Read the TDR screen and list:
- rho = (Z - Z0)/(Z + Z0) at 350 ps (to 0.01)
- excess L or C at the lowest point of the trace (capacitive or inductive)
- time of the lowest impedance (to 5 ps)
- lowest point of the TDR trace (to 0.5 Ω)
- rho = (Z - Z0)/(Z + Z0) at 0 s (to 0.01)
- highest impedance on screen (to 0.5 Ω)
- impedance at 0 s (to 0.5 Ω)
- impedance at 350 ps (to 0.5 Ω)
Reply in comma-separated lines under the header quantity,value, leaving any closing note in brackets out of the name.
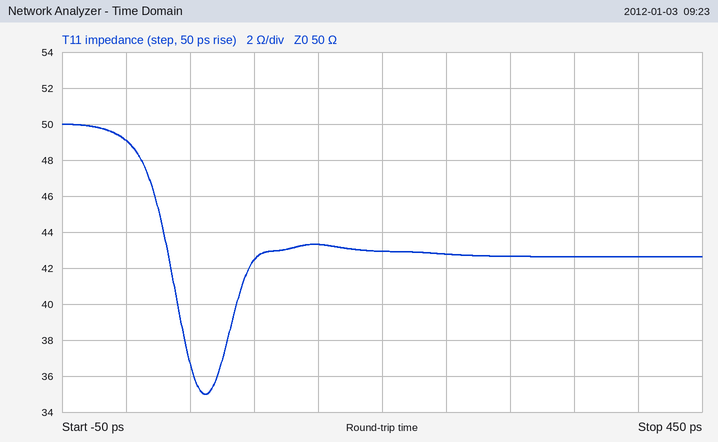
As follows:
quantity,value
rho = (Z - Z0)/(Z + Z0) at 350 ps,-0.08
excess L or C at the lowest point of the trace,capacitive
time of the lowest impedance,60 ps
lowest point of the TDR trace,35.0 Ω
rho = (Z - Z0)/(Z + Z0) at 0 s,-0.01
highest impedance on screen,50.0 Ω
impedance at 0 s,49.0 Ω
impedance at 350 ps,42.5 Ω
